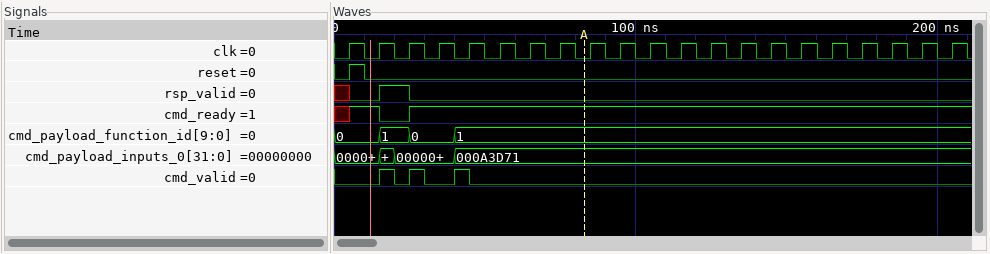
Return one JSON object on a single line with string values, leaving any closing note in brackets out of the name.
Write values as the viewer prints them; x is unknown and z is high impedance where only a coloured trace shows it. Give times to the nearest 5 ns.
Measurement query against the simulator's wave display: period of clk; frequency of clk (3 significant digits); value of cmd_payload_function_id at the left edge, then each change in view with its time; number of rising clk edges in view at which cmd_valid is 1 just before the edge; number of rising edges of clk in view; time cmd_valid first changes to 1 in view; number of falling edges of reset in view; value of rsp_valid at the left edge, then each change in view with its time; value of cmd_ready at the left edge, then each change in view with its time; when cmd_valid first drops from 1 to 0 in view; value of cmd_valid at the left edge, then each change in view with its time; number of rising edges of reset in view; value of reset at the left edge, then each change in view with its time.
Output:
{"period of clk": "10 ns", "frequency of clk": "100 MHz", "value of cmd_payload_function_id at the left edge, then each change in view with its time": "0, 1 at 15 ns, 0 at 25 ns, 1 at 40 ns", "number of rising clk edges in view at which cmd_valid is 1 just before the edge": "1", "number of rising edges of clk in view": "21", "time cmd_valid first changes to 1 in view": "15 ns", "number of falling edges of reset in view": "1", "value of rsp_valid at the left edge, then each change in view with its time": "x, 0 at 5 ns, 1 at 15 ns, 0 at 25 ns", "value of cmd_ready at the left edge, then each change in view with its time": "x, 1 at 5 ns, 0 at 15 ns, 1 at 25 ns", "when cmd_valid first drops from 1 to 0 in view": "20 ns", "value of cmd_valid at the left edge, then each change in view with its time": "0, 1 at 15 ns, 0 at 20 ns, 1 at 25 ns, 0 at 30 ns, 1 at 40 ns, 0 at 45 ns", "number of rising edges of reset in view": "1", "value of reset at the left edge, then each change in view with its time": "0, 1 at 5 ns, 0 at 10 ns"}
